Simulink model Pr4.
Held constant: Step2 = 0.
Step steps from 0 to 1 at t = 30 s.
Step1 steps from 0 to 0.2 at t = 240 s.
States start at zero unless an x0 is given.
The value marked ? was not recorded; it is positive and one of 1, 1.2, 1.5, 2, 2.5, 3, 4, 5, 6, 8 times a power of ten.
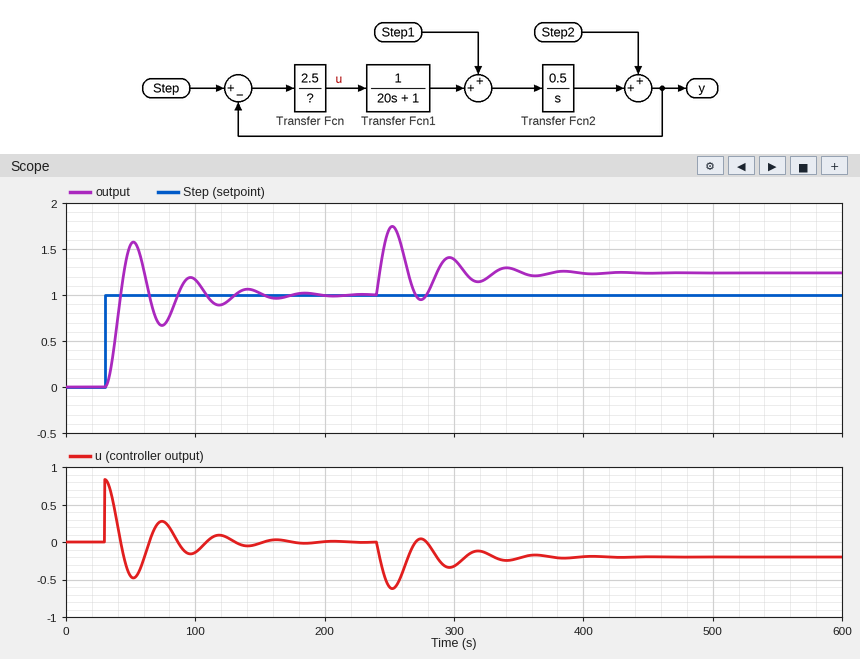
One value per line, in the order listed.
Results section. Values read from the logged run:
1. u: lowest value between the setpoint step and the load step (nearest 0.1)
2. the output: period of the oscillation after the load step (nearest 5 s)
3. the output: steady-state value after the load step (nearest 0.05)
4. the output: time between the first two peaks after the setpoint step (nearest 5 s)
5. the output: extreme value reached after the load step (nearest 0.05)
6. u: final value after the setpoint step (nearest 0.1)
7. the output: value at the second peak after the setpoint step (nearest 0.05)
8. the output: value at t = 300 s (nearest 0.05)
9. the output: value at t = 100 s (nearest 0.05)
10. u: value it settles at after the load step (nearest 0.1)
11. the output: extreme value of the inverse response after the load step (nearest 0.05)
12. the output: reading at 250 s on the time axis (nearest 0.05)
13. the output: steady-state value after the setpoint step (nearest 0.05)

-0.5
45 s
1.25
45 s
1.75
0.0
1.20
1.40
1.15
-0.2
0.95
1.70
1.00
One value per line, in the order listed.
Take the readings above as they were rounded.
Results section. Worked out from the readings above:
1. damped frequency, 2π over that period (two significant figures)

0.14 rad/s
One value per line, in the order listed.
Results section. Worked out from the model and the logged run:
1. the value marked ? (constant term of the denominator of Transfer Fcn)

3
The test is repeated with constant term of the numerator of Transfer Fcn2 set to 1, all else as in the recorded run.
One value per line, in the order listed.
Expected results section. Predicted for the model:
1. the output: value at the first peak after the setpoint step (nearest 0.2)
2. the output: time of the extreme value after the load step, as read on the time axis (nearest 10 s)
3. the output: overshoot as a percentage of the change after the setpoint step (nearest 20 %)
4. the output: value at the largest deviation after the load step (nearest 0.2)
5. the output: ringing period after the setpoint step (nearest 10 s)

1.6
250 s
60 %
2.0
30 s
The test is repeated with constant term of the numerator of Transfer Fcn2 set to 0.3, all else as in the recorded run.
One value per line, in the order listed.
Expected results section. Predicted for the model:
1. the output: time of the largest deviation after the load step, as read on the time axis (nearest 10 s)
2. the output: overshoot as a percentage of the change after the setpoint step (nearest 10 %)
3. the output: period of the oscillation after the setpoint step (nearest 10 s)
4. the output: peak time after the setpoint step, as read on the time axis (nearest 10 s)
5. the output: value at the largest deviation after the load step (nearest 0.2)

260 s
50 %
60 s
60 s
1.6
